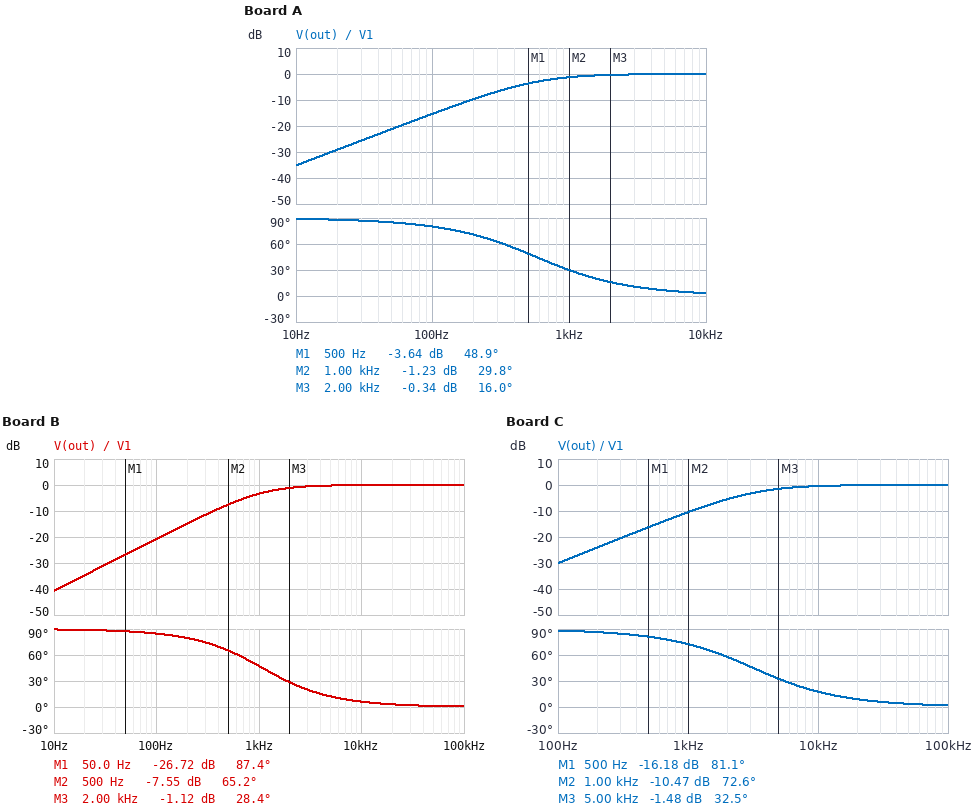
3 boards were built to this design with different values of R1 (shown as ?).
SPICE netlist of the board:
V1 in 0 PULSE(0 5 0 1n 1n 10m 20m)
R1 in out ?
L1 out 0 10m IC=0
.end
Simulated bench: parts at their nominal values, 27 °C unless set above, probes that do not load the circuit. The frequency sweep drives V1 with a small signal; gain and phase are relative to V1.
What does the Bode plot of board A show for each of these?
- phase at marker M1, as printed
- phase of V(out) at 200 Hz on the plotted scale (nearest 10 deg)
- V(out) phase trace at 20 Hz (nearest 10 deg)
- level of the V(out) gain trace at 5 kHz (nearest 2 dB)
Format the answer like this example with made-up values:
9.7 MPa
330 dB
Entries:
48.9 deg
70 deg
90 deg
0 dB
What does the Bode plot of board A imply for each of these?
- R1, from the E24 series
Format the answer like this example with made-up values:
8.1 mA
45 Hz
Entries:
36 Ω
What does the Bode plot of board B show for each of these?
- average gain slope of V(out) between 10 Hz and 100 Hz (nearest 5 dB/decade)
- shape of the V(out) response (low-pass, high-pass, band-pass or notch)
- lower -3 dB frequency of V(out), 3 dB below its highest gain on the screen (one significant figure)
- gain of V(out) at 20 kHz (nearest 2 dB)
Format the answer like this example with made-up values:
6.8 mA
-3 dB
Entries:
20 dB/decade
high-pass
1 kHz
0 dB
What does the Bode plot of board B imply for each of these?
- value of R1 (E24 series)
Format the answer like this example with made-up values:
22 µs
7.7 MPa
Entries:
68 Ω
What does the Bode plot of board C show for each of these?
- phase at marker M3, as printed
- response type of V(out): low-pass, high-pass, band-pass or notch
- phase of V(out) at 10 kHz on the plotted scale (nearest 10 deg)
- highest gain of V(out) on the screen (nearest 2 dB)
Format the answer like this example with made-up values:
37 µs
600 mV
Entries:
32.5 deg
high-pass
20 deg
0 dB
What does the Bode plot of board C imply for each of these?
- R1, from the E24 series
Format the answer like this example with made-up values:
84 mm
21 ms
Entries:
200 Ω
